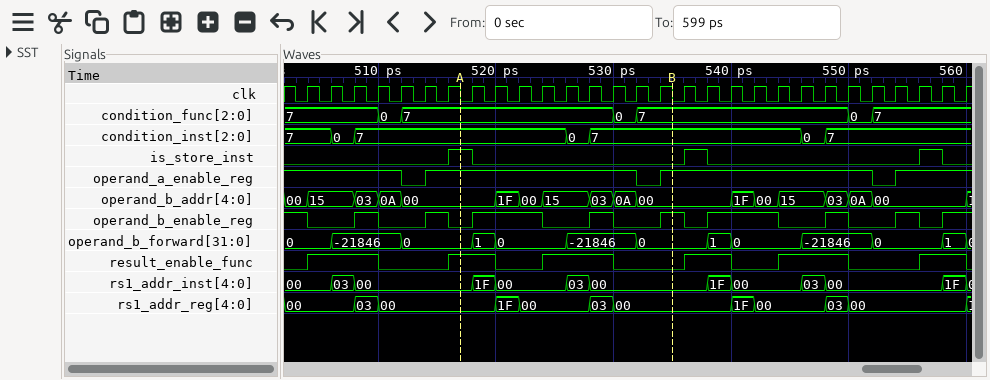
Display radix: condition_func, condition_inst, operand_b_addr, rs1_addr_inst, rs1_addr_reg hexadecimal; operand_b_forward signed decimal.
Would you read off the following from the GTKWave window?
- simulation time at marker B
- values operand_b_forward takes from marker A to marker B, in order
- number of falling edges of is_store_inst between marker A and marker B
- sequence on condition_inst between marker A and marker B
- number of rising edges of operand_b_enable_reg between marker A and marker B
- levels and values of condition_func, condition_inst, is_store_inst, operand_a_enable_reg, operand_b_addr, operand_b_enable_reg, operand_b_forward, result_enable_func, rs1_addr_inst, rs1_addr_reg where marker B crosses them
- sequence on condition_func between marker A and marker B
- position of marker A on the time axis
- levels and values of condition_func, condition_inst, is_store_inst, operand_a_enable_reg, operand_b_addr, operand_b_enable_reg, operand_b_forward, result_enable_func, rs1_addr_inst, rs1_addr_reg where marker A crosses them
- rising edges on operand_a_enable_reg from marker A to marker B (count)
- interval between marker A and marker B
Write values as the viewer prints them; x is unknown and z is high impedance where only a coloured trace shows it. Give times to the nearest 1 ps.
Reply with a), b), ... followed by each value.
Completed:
a) 535 ps
b) 0, 1, 0, -21846, 0
c) 1
d) 7, 0, 7
e) 3
f) condition_func=7, condition_inst=7, is_store_inst=0, operand_a_enable_reg=1, operand_b_addr=00, operand_b_enable_reg=1, operand_b_forward=0, result_enable_func=0, rs1_addr_inst=00, rs1_addr_reg=00
g) 7, 0, 7
h) 517 ps
i) condition_func=7, condition_inst=7, is_store_inst=1, operand_a_enable_reg=1, operand_b_addr=00, operand_b_enable_reg=0, operand_b_forward=0, result_enable_func=1, rs1_addr_inst=00, rs1_addr_reg=00
j) 1
k) 18 ps
